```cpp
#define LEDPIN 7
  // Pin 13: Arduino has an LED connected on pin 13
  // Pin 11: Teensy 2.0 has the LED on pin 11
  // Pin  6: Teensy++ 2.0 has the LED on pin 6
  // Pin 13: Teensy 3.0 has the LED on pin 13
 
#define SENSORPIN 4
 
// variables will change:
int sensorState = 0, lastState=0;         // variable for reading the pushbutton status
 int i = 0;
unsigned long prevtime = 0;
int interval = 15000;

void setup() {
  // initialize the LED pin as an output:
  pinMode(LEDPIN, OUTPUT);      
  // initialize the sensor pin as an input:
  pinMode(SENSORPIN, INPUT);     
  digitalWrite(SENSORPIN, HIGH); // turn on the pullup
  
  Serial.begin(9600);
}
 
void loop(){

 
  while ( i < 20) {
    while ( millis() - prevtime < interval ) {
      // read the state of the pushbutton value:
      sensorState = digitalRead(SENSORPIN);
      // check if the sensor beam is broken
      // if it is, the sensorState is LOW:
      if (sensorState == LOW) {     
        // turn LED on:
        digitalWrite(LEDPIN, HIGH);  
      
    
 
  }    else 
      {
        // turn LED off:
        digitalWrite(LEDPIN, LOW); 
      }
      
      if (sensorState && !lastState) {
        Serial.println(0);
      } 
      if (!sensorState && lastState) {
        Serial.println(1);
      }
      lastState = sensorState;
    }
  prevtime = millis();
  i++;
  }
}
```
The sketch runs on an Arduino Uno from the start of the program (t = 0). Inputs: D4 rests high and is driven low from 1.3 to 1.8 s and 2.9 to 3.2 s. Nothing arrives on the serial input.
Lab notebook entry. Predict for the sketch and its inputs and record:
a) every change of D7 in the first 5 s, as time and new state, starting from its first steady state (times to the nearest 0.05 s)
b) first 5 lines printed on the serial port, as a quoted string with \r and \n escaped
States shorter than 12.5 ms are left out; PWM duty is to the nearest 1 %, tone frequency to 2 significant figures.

0 s low; 1.3 s high; 1.8 s low; 2.9 s high; 3.2 s low
"0\r\n1\r\n0\r\n1\r\n0\r\n"
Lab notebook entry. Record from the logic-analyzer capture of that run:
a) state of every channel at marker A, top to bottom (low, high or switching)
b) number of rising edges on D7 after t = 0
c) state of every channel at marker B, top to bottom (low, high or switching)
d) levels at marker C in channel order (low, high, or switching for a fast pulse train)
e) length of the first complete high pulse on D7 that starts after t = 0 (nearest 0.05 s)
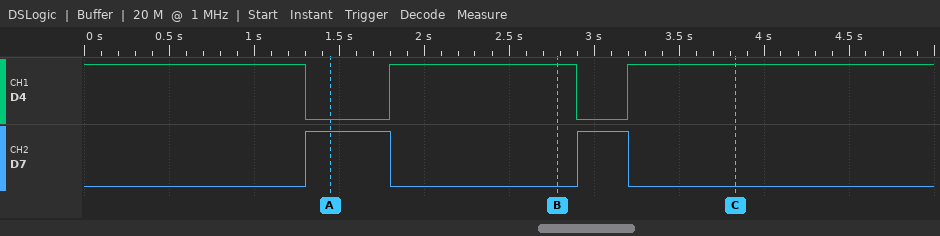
D4 low, D7 high
2
D4 high, D7 low
D4 high, D7 low
0.50 s
